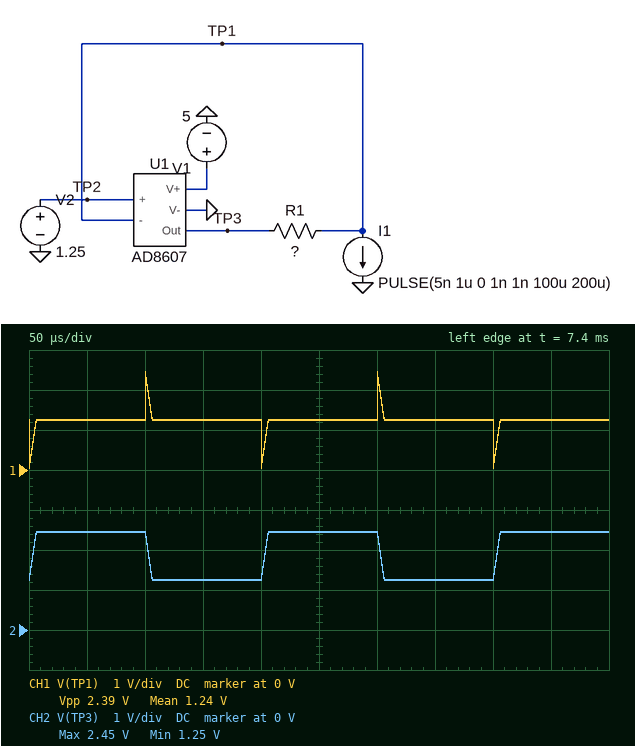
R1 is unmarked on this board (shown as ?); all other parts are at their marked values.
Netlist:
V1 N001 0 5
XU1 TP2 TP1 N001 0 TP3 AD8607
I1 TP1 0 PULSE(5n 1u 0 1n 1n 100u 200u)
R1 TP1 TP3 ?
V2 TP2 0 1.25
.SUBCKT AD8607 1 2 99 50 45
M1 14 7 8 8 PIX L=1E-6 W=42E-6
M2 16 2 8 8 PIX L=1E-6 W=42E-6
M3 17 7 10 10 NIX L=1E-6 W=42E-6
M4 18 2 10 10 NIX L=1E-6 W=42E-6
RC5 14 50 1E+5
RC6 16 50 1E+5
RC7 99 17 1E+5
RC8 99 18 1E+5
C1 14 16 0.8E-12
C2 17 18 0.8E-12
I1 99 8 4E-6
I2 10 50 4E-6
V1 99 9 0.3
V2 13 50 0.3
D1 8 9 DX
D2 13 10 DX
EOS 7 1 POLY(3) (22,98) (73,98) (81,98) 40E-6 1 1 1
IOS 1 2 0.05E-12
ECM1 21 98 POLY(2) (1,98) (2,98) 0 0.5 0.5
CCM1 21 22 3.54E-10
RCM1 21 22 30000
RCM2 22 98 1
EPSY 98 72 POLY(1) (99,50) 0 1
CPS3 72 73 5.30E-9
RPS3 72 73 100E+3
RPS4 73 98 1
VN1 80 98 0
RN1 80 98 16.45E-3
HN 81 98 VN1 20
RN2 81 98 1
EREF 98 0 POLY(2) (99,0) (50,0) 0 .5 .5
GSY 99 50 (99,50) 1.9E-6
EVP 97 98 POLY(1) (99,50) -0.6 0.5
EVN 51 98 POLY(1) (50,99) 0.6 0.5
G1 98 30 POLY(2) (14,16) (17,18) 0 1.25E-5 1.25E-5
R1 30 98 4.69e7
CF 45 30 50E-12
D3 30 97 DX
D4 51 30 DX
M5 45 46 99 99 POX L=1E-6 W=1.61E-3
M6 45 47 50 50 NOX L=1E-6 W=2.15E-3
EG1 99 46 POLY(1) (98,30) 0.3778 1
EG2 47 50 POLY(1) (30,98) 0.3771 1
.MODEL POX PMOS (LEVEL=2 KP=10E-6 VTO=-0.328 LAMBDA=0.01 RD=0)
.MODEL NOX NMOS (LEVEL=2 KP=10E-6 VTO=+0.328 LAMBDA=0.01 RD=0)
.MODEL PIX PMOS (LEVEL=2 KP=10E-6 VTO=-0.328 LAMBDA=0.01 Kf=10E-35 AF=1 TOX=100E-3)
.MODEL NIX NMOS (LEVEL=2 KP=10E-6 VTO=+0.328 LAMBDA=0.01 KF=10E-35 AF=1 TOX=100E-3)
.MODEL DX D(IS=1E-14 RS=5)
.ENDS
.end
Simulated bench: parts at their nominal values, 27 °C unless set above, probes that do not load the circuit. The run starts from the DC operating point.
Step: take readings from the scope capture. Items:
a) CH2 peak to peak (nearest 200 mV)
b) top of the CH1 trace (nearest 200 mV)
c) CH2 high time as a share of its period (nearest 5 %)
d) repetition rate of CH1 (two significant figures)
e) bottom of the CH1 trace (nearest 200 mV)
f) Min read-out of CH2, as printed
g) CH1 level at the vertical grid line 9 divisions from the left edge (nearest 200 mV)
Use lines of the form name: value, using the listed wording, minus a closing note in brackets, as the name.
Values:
CH2 peak to peak: 1.2 V
top of the CH1 trace: 2.4 V
CH2 high time as a share of its period: 50 %
repetition rate of CH1: 5.0 kHz
bottom of the CH1 trace: 0 V
Min read-out of CH2, as printed: 1.25 V
CH1 level at the vertical grid line 9 divisions from the left edge: 1.2 V
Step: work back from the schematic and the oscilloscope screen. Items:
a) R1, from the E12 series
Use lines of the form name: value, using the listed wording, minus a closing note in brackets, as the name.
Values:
R1, from the E12 series: 1.2 MΩ
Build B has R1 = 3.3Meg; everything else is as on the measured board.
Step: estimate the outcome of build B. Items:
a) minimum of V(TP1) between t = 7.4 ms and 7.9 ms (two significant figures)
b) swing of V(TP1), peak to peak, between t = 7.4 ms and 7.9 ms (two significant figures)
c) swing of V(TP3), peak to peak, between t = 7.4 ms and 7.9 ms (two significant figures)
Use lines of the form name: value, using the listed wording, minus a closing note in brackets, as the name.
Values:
minimum of V(TP1) between t = 7.4 ms and 7.9 ms: -2.0 V
swing of V(TP1), peak to peak, between t = 7.4 ms and 7.9 ms: 6.6 V
swing of V(TP3), peak to peak, between t = 7.4 ms and 7.9 ms: 3.3 V
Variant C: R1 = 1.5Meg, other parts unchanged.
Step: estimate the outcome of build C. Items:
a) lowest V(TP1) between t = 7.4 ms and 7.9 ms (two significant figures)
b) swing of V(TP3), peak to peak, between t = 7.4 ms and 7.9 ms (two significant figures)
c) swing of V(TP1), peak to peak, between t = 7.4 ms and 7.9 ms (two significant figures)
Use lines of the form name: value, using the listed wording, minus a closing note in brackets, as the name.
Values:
lowest V(TP1) between t = 7.4 ms and 7.9 ms: -240 mV
swing of V(TP3), peak to peak, between t = 7.4 ms and 7.9 ms: 1.5 V
swing of V(TP1), peak to peak, between t = 7.4 ms and 7.9 ms: 3.0 V
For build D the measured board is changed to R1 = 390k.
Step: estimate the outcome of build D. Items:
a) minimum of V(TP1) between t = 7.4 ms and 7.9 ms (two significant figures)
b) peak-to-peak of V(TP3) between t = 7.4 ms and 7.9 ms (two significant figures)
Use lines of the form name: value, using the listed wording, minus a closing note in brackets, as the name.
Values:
minimum of V(TP1) between t = 7.4 ms and 7.9 ms: 860 mV
peak-to-peak of V(TP3) between t = 7.4 ms and 7.9 ms: 390 mV
